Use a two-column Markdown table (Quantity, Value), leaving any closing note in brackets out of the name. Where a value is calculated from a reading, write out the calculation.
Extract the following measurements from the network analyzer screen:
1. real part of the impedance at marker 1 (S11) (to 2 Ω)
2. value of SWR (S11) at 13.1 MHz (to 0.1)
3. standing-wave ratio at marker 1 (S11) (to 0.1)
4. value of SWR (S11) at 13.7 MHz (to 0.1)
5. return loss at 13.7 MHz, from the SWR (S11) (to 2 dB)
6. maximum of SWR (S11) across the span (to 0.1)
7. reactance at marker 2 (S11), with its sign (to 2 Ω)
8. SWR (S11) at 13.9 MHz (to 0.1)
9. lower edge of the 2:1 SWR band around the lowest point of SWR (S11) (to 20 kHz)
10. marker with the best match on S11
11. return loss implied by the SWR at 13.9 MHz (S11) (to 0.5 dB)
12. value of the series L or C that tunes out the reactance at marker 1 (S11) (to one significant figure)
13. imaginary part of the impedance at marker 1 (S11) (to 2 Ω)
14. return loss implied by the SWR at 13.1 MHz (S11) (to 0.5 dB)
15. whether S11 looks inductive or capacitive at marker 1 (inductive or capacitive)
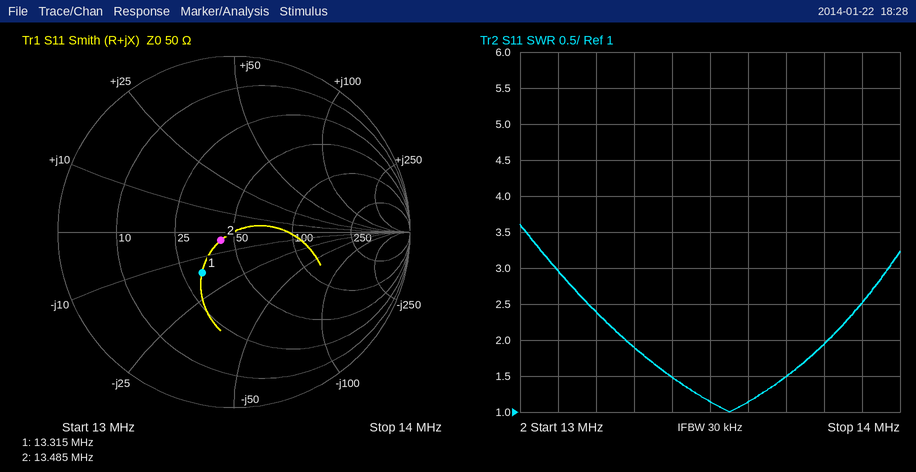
| Quantity | Value |
|---|---|
| real part of the impedance at marker 1 (S11) | 32 Ω |
| value of SWR (S11) at 13.1 MHz | 3.0 |
| standing-wave ratio at marker 1 (S11) | 1.8 |
| value of SWR (S11) at 13.7 MHz | 1.5 |
| return loss at 13.7 MHz, from the SWR (S11) | −20 log10((1.5 − 1)/(1.5 + 1)) ≈ 14 dB |
| maximum of SWR (S11) across the span | 3.6 |
| reactance at marker 2 (S11), with its sign | -4 Ω |
| SWR (S11) at 13.9 MHz | 2.5 |
| lower edge of the 2:1 SWR band around the lowest point of SWR (S11) | 13.28 MHz |
| marker with the best match on S11 | marker 2 |
| return loss implied by the SWR at 13.9 MHz (S11) | −20 log10((2.5 − 1)/(2.5 + 1)) ≈ 7.36 dB, so 7.5 dB to the nearest 0.5 dB |
| value of the series L or C that tunes out the reactance at marker 1 (S11) | L = 16 Ω/(2π × 13.315 MHz) ≈ 191 nH, so 200 nH to one significant figure |
| imaginary part of the impedance at marker 1 (S11) | -16 Ω |
| return loss implied by the SWR at 13.1 MHz (S11) | −20 log10((3 − 1)/(3 + 1)) ≈ 6.0 dB |
| whether S11 looks inductive or capacitive at marker 1 | capacitive |
